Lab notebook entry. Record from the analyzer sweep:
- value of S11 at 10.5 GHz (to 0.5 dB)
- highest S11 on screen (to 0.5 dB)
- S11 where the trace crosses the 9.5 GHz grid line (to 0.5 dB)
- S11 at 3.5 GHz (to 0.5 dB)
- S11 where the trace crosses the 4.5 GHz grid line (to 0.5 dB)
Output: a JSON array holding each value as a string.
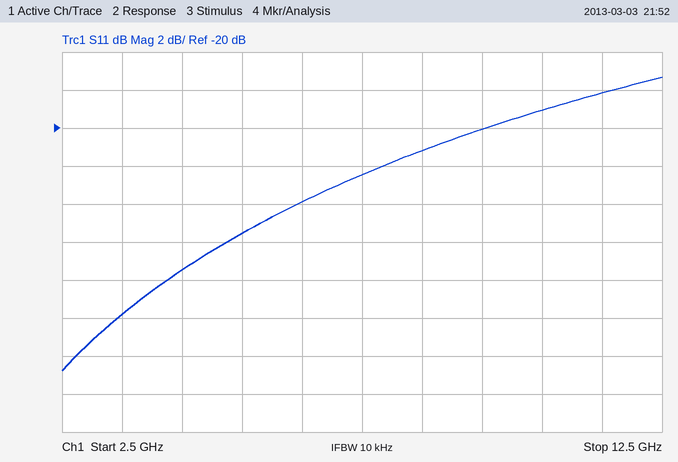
["-19.0 dB", "-17.5 dB", "-20.0 dB", "-30.0 dB", "-27.5 dB"]
